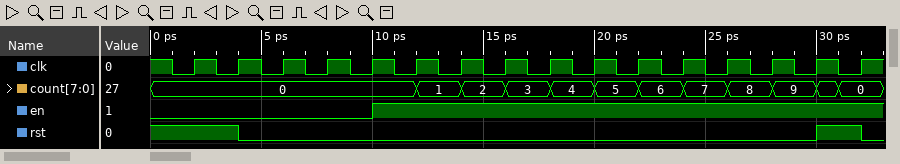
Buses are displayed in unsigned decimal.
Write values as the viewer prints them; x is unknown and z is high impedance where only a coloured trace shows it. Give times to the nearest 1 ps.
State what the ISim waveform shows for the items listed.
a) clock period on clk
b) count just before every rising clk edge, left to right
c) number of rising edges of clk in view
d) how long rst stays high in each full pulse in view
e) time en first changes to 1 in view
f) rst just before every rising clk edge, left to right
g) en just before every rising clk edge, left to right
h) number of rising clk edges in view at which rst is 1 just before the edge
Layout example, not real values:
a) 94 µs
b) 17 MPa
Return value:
a) 2 ps
b) 0, 0, 0, 0, 0, 0, 1, 2, 3, 4, 5, 6, 7, 8, 9, 0
c) 16
d) 2 ps
e) 10 ps
f) 1 1 0 0 0 0 0 0 0 0 0 0 0 0 0 1
g) 0 0 0 0 0 1 1 1 1 1 1 1 1 1 1 1
h) 3
